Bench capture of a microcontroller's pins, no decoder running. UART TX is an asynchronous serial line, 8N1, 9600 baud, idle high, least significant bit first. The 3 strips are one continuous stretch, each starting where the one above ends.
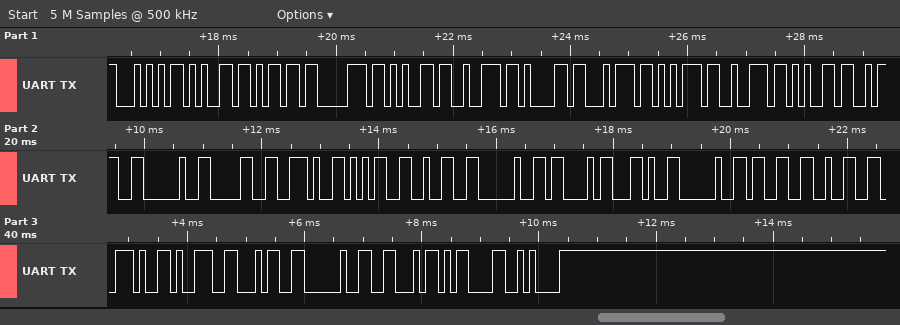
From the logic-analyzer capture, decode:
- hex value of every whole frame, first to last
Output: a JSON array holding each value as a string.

["54 65 6D 70 65 72 61 74 75 72 65 3A 20 30 2E 35 32 20 43 2C 20 33 32 2E 39 34 20 46 0D 0A"]
